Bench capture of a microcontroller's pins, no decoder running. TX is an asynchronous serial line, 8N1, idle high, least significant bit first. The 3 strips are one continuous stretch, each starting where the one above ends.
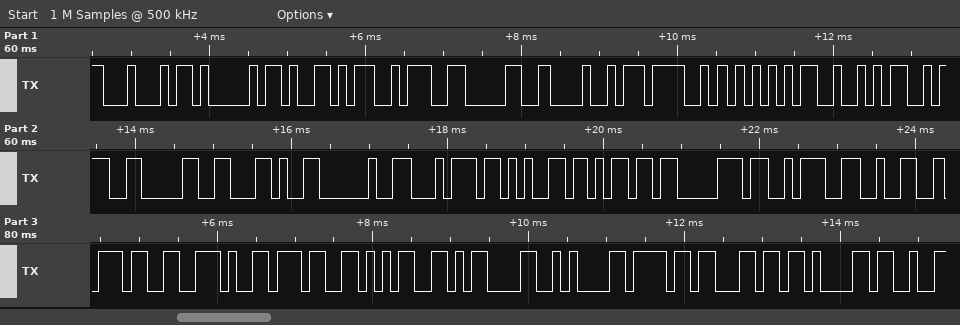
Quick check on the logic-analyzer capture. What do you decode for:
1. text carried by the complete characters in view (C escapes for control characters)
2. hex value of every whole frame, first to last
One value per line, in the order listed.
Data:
"DAY:0HOUR:0, temp:27.75\r\nola"
0x44 0x41 0x59 0x3A 0x30 0x48 0x4F 0x55 0x52 0x3A 0x30 0x2C 0x20 0x74 0x65 0x6D 0x70 0x3A 0x32 0x37 0x2E 0x37 0x35 0x0D 0x0A 0x6F 0x6C 0x61
